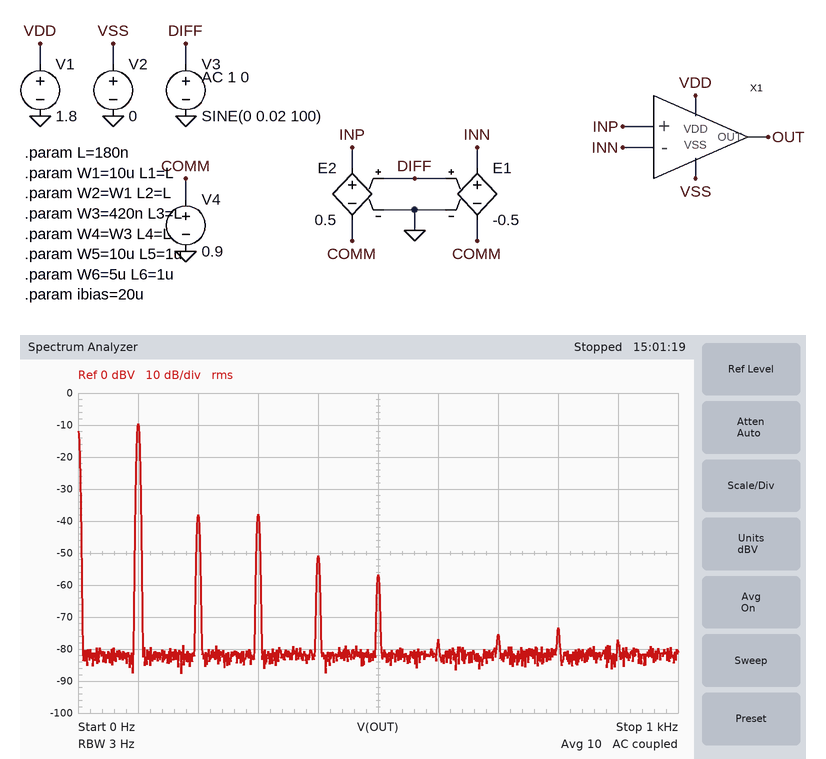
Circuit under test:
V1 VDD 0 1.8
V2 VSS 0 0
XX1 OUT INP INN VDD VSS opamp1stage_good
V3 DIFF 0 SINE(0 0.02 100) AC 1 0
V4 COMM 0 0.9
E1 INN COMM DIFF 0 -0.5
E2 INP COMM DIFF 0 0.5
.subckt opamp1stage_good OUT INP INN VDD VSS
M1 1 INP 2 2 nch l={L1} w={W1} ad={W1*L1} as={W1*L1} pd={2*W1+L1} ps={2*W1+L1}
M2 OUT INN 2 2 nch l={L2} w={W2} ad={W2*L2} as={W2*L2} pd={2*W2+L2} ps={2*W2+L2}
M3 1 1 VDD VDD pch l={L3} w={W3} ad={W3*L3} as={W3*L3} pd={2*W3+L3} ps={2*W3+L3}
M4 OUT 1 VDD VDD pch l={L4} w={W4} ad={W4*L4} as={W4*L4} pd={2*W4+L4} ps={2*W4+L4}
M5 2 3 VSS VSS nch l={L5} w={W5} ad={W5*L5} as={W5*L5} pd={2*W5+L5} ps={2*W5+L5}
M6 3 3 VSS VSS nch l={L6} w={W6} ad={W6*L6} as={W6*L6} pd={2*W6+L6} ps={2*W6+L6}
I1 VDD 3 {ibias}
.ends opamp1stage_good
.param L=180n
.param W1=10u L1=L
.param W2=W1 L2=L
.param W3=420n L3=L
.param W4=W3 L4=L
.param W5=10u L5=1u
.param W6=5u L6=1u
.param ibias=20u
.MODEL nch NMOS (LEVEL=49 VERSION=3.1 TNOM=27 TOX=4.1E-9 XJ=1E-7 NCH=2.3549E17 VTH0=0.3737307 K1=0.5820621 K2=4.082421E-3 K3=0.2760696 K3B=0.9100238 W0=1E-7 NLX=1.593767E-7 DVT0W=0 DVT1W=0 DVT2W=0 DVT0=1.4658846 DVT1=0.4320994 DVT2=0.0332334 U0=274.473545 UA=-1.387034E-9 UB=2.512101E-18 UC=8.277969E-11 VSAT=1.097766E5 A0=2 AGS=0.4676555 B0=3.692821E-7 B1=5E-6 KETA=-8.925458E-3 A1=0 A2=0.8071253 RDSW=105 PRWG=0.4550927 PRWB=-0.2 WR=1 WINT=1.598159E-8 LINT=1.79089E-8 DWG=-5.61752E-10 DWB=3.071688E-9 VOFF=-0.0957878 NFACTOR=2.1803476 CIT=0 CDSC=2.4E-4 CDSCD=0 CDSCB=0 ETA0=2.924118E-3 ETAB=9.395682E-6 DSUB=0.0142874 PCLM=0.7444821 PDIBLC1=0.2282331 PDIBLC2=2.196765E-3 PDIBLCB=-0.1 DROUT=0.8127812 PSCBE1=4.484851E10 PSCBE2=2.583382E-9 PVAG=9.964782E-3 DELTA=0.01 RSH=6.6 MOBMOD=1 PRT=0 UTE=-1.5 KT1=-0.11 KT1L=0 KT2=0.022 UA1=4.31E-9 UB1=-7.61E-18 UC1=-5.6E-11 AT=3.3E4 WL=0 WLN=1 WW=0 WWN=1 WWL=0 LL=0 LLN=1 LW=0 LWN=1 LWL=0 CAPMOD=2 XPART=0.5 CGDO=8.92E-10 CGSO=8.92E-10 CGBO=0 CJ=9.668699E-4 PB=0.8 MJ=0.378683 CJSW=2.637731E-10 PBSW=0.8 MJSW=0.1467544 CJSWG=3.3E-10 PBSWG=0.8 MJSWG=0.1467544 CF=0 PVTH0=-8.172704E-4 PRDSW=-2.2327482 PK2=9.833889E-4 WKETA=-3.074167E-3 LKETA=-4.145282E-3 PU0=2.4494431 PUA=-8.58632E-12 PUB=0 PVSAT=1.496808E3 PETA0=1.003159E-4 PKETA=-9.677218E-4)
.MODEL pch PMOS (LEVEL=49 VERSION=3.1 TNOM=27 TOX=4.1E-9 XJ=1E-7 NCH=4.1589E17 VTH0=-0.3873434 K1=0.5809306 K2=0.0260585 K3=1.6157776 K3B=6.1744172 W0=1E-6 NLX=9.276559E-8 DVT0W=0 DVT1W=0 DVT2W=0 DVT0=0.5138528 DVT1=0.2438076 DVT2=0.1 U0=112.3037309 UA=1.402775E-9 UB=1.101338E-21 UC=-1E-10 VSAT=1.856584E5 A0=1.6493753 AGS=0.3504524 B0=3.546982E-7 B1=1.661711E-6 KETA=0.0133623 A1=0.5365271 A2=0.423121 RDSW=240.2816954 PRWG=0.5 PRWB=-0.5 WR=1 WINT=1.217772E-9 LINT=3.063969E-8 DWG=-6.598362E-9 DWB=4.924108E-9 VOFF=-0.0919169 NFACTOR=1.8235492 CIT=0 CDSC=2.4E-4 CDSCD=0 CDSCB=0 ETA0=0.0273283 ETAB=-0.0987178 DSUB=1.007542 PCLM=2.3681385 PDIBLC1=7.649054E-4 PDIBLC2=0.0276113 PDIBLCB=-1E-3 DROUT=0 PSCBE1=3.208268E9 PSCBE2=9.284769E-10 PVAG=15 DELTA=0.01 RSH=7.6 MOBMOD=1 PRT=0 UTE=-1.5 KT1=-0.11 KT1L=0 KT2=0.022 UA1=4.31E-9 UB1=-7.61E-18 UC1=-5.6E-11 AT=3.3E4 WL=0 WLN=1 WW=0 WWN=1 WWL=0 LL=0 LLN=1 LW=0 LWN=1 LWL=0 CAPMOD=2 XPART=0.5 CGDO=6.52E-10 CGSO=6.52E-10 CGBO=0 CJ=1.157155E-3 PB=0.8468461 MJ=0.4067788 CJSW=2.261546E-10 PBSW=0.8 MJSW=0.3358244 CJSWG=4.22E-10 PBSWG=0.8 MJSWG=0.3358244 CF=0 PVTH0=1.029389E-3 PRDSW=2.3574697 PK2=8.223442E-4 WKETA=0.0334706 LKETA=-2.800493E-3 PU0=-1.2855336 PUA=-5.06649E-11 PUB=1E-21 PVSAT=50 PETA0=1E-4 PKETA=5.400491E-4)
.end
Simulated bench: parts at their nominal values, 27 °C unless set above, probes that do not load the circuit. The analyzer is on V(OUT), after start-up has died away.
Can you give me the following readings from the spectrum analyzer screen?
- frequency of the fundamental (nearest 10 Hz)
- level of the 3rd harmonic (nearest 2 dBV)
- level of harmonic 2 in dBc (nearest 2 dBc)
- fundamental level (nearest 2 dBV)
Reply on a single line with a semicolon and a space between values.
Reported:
100 Hz; -38 dBV; -28 dBc; -10 dBV
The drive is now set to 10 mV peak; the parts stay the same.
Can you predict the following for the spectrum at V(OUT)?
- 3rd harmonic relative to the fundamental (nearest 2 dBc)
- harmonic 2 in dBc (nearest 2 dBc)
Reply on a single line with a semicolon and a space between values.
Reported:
-46 dBc; -44 dBc
